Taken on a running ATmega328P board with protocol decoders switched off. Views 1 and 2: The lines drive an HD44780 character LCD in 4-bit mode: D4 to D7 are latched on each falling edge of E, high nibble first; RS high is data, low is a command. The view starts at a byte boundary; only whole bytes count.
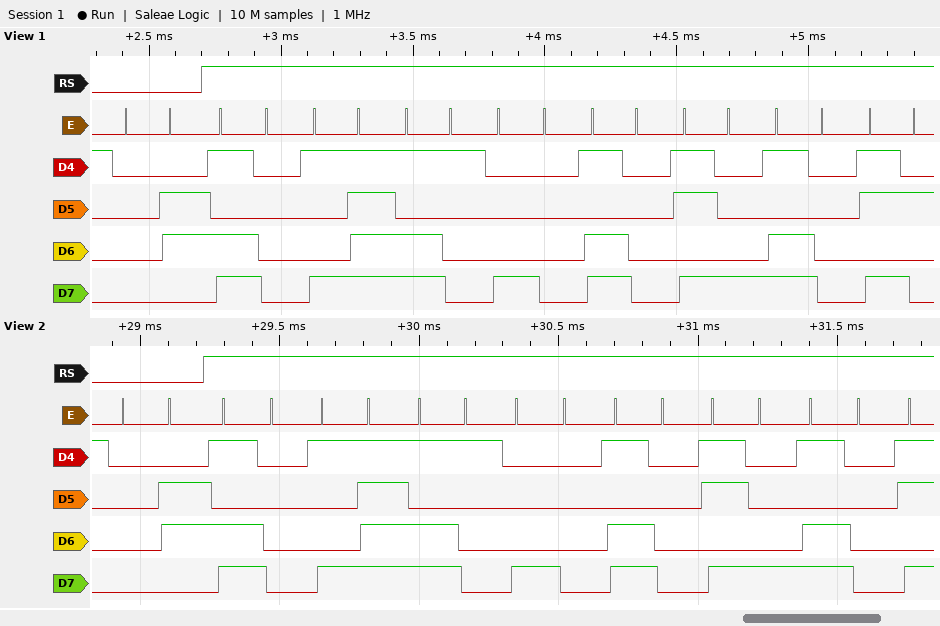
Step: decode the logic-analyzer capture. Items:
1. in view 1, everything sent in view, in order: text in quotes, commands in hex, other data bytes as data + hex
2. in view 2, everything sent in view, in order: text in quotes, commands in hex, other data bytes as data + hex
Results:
0x06 data D0 9F D1 80 D0 B8 D0 B2
0x06 data D0 9F D1 80 D0 B8 D0
